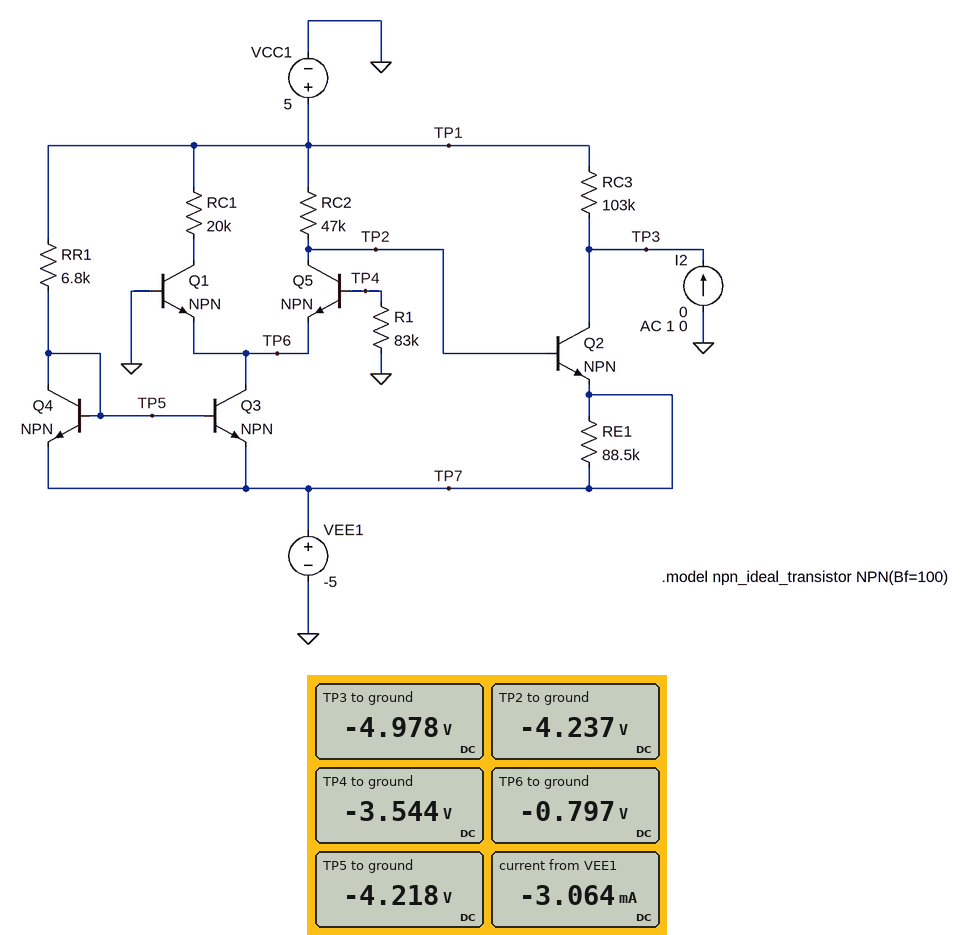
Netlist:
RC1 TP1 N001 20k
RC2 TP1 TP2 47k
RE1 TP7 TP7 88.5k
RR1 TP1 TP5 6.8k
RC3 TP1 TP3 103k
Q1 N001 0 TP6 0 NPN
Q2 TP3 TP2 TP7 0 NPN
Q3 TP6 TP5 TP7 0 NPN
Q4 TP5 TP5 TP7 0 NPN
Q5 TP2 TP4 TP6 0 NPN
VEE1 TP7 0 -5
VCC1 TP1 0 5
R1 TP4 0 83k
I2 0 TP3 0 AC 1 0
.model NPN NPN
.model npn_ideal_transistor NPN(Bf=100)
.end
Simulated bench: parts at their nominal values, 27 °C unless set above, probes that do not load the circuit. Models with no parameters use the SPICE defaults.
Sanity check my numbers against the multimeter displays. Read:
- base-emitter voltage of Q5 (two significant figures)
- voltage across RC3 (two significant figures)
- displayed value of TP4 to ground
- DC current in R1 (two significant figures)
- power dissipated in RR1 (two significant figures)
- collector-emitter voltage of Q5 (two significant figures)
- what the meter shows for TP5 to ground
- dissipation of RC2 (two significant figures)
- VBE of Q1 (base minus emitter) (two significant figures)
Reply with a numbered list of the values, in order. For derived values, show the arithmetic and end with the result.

1. -3.544 V - (-797 mV) = -2.7 V
2. 5 V - (-4.978 V) = 10 V
3. -3.544 V
4. (0 V - (-3.544 V)) / 83 kΩ = 43 µA
5. (5 V - (-4.218 V))^2 / 6.8 kΩ = 12 mW
6. -4.237 V - (-797 mV) = -3.4 V
7. -4.218 V
8. (5 V - (-4.237 V))^2 / 47 kΩ = 1.8 mW
9. 0 V - (-797 mV) = 800 mV
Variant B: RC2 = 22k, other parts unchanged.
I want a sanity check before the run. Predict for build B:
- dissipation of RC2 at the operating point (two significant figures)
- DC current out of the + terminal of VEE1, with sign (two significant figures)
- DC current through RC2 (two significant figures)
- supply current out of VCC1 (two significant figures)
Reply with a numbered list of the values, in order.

1. 3.9 mW
2. -3.3 mA
3. 420 µA
4. 2.2 mA
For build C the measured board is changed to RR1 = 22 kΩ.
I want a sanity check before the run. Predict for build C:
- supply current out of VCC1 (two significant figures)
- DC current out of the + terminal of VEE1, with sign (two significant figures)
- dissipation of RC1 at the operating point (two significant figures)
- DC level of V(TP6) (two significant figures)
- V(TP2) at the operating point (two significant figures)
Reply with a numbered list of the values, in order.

1. 1.0 mA
2. -1.2 mA
3. 1.6 mW
4. -760 mV
5. -4.2 V
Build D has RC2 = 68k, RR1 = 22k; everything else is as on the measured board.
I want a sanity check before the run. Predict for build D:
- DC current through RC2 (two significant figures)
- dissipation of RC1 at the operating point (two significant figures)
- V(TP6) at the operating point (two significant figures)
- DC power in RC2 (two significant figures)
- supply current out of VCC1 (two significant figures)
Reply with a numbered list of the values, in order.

1. 140 µA
2. 1.6 mW
3. -760 mV
4. 1.3 mW
5. 940 µA
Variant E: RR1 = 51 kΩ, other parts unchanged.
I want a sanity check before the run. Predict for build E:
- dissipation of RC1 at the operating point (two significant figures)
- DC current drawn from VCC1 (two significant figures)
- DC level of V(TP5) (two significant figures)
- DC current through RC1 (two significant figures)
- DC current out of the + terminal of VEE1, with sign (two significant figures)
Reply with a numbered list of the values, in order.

1. 960 µW
2. 690 µA
3. -4.3 V
4. 220 µA
5. -740 µA
